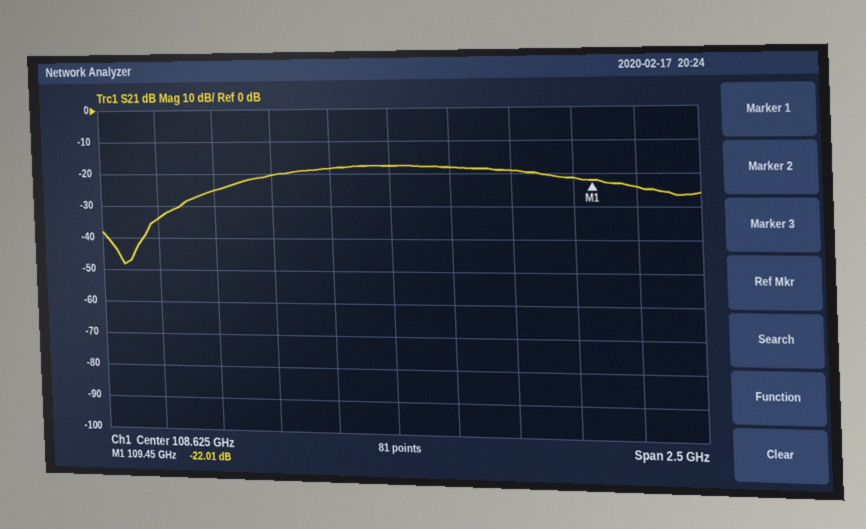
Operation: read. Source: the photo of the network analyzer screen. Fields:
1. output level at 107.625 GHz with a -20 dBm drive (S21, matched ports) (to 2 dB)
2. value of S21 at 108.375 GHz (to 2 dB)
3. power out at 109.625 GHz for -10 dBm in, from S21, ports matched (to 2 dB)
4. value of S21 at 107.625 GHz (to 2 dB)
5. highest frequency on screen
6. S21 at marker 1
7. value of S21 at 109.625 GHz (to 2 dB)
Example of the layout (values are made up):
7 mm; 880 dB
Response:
-54 dBm; -18 dB; -34 dBm; -34 dB; 109.875 GHz; -22.01 dB; -24 dB
